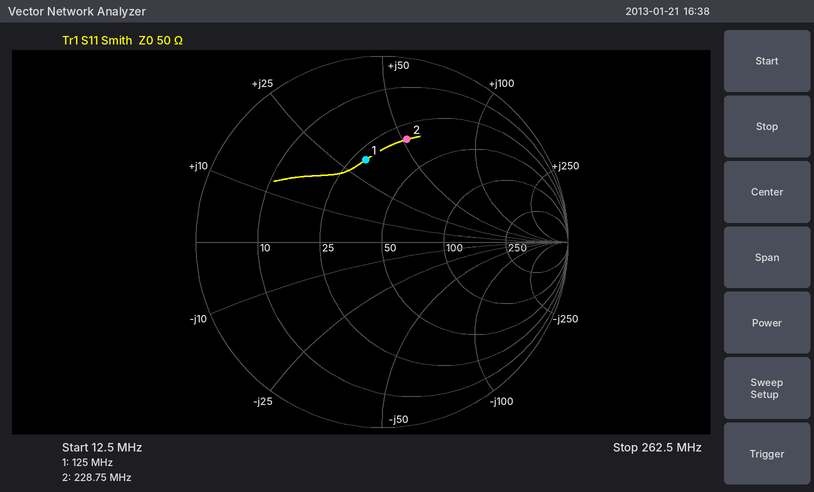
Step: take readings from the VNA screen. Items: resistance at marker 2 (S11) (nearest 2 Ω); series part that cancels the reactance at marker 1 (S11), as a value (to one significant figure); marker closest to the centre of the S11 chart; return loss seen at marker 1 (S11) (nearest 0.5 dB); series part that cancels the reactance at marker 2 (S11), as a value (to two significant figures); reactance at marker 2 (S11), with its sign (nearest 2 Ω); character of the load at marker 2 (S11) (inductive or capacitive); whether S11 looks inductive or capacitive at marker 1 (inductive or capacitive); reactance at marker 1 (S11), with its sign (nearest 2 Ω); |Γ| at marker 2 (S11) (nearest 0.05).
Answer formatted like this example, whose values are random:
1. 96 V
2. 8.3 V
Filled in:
1. 32 Ω
2. 40 pF
3. marker 1
4. 7.0 dB
5. 13 pF
6. +52 Ω
7. inductive
8. inductive
9. +32 Ω
10. 0.55
